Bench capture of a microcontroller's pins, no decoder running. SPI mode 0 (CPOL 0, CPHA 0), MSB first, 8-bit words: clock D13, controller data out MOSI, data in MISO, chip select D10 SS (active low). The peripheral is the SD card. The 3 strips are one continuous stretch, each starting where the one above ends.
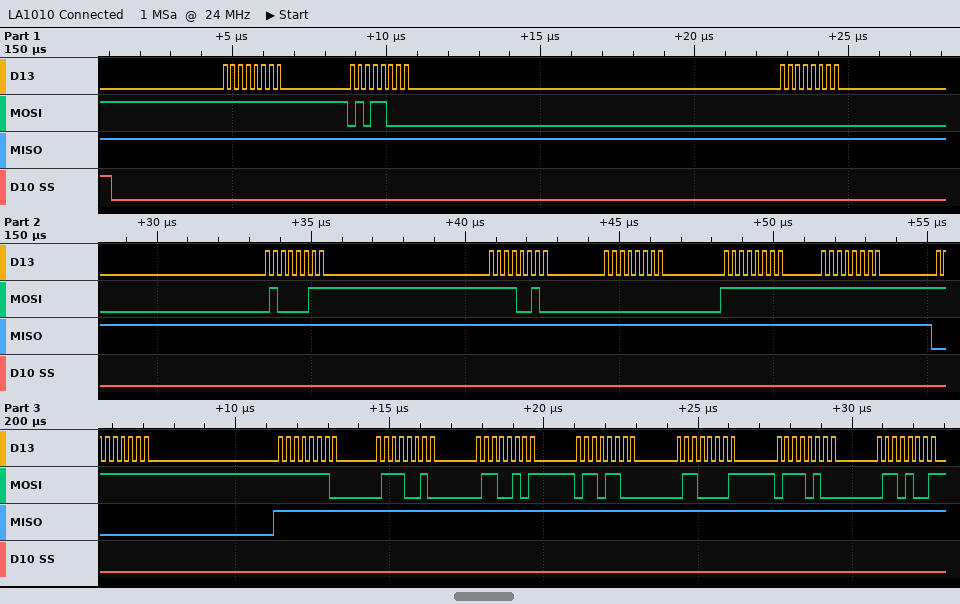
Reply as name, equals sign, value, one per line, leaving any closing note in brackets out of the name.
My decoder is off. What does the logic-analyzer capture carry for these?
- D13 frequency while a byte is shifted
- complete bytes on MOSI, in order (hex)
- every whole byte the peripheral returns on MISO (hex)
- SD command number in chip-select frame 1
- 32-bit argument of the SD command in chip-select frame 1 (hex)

D13 frequency while a byte is shifted = 4 MHz
complete bytes on MOSI, in order = FF 58 00 43 F2 00 FF FF FF FE 72 65 6C 61 74 69
every whole byte the peripheral returns on MISO = FF FF FF FF FF FF FF FF 00 FF FF FF FF FF FF FF
SD command number in chip-select frame 1 = CMD24
32-bit argument of the SD command in chip-select frame 1 = 0x0043F200
